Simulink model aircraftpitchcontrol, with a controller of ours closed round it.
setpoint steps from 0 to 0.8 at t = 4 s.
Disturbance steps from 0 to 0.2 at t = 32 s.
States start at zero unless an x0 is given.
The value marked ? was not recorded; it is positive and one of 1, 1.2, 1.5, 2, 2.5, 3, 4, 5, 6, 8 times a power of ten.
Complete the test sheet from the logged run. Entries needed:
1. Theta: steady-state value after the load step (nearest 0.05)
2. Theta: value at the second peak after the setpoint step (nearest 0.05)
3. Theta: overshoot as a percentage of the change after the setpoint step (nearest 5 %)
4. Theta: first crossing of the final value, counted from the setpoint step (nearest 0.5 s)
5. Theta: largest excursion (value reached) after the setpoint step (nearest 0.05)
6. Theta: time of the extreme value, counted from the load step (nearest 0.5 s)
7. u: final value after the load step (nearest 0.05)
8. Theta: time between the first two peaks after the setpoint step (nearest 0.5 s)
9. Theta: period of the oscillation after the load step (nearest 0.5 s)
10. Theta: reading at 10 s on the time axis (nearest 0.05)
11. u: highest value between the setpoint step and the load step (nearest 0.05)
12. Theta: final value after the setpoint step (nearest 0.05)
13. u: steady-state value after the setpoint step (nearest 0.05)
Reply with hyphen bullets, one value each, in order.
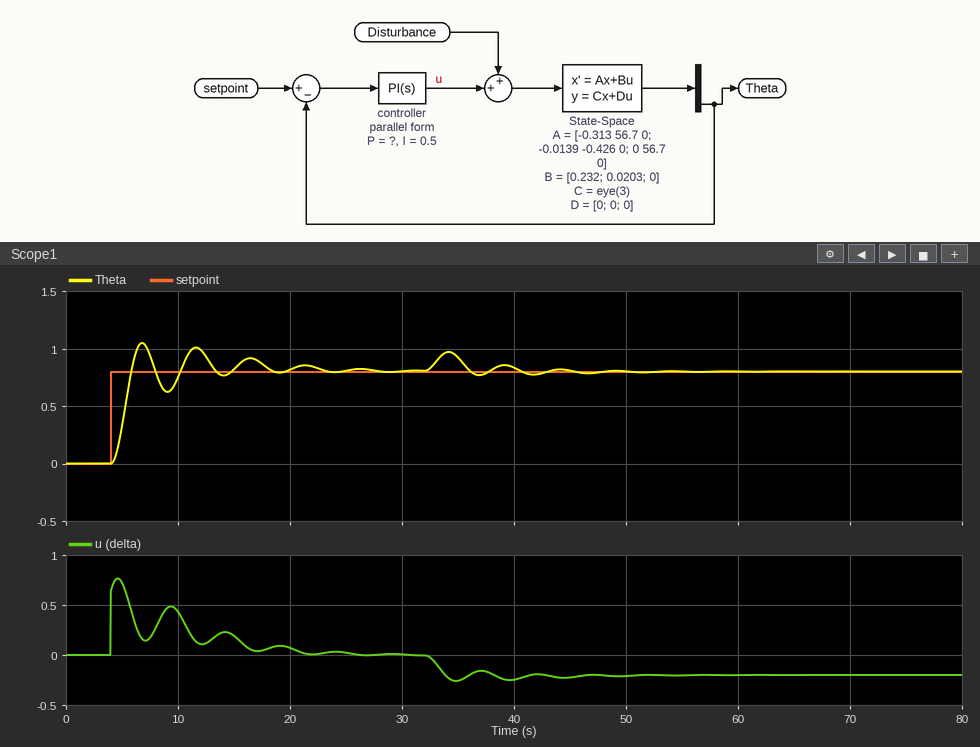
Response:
- 0.80
- 1.00
- 30 %
- 2.0 s
- 1.05
- 2.0 s
- -0.20
- 5.0 s
- 5.0 s
- 0.75
- 0.75
- 0.80
- 0.00
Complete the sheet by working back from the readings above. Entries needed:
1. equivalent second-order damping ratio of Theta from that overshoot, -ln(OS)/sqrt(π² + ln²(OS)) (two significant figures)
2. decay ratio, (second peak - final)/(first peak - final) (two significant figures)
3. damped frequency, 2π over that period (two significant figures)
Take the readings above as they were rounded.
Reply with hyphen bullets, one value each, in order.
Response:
- 0.36
- 0.80
- 1.3 rad/s
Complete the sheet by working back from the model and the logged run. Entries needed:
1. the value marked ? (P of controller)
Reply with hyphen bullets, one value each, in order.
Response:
- 0.8
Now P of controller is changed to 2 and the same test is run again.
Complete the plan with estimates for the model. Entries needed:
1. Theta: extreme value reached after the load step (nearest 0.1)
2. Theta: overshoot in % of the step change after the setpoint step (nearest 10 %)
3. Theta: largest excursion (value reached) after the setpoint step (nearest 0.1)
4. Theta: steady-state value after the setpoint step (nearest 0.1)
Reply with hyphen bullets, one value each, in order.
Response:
- 0.9
- 40 %
- 1.1
- 0.8
